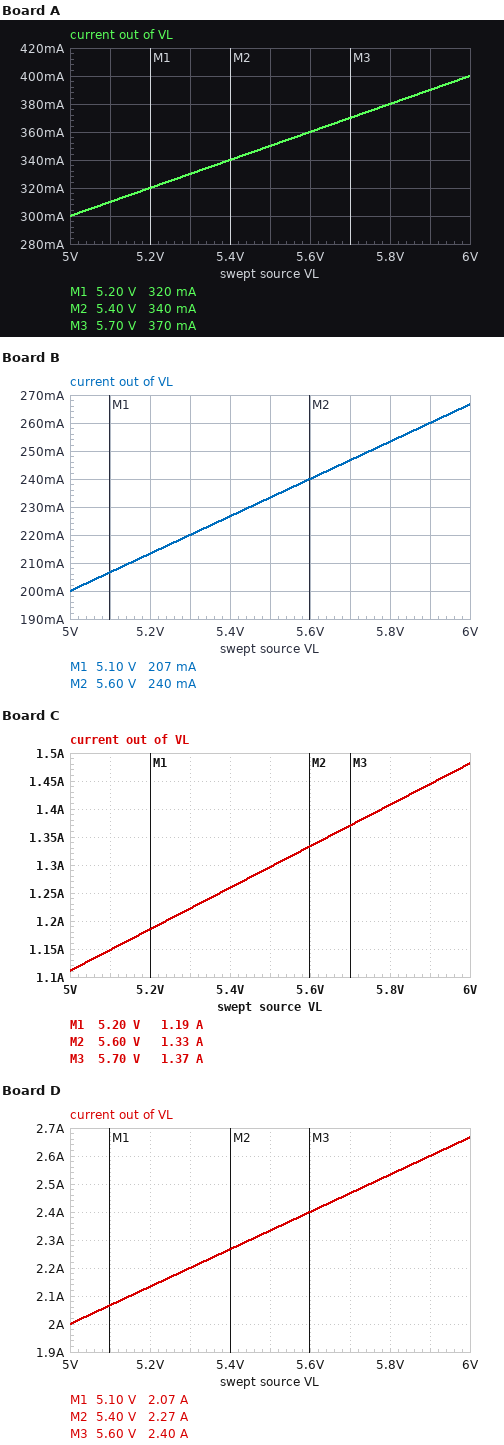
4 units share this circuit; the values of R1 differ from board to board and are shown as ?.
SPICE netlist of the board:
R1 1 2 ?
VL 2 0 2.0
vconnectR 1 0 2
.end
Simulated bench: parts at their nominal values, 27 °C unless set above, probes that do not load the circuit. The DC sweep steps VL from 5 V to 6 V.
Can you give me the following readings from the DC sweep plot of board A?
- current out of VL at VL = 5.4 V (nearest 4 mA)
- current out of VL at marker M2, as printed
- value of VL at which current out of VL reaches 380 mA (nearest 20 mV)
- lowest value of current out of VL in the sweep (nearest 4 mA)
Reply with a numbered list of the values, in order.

1. 340 mA
2. 340 mA
3. 5.80 V
4. 300 mA
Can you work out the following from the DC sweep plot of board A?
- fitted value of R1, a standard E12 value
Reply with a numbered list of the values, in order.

1. 10 Ω
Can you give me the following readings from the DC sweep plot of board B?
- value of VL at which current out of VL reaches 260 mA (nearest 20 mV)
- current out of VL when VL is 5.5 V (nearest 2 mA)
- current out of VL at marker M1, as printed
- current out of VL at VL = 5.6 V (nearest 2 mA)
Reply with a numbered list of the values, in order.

1. 5.90 V
2. 234 mA
3. 207 mA
4. 240 mA
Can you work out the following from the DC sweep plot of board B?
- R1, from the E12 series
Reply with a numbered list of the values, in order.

1. 15 Ω
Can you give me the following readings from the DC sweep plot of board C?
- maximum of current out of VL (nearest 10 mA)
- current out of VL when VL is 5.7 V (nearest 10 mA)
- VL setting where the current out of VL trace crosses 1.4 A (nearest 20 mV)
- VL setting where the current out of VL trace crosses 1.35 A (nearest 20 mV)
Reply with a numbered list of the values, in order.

1. 1.48 A
2. 1.37 A
3. 5.78 V
4. 5.64 V
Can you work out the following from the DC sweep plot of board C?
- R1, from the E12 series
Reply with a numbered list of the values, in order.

1. 2.7 Ω
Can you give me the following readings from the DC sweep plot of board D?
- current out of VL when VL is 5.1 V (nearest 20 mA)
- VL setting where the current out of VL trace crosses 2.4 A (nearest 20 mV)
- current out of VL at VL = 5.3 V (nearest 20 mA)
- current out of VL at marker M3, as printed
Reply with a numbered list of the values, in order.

1. 2.06 A
2. 5.60 V
3. 2.20 A
4. 2.40 A
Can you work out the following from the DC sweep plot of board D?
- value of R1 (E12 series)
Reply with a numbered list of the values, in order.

1. 1.5 Ω
